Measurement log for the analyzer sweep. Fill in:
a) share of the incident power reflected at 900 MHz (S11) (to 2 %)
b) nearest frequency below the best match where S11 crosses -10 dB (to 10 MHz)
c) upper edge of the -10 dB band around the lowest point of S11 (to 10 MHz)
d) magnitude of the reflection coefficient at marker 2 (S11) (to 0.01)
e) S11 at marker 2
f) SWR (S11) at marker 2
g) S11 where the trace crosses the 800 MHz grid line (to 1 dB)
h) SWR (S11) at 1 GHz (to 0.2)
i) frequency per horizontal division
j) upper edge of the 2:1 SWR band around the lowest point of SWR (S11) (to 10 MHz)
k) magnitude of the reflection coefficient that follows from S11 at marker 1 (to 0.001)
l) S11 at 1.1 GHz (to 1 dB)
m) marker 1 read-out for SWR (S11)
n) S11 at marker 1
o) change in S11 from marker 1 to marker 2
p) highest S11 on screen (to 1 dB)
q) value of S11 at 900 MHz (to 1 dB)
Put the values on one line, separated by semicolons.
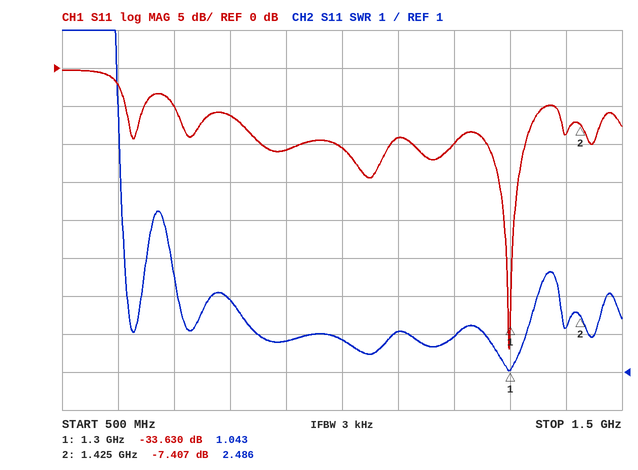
8 %; 1.26 GHz; 1.33 GHz; 0.43; -7.407 dB; 2.486; -6 dB; 1.8; 100 MHz; 1.33 GHz; 0.021; -9 dB; 1.043; -33.630 dB; 26.223 dB; 0 dB; -11 dB
